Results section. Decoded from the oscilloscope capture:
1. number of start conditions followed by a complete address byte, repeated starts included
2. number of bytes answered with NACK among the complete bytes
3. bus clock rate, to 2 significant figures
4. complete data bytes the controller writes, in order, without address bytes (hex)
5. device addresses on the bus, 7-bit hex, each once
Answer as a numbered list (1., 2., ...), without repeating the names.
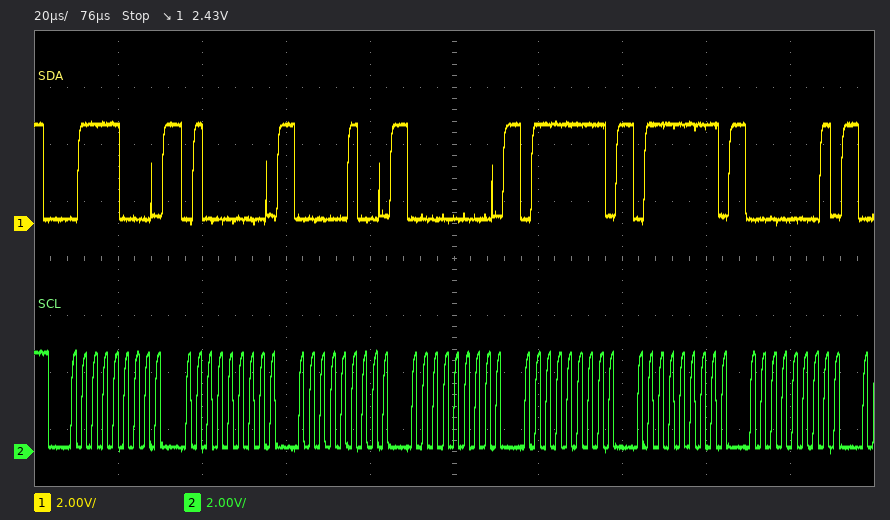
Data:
1. 1
2. 0
3. 400 kHz
4. 40 04 00 7F 7F 01
5. 0x3C
